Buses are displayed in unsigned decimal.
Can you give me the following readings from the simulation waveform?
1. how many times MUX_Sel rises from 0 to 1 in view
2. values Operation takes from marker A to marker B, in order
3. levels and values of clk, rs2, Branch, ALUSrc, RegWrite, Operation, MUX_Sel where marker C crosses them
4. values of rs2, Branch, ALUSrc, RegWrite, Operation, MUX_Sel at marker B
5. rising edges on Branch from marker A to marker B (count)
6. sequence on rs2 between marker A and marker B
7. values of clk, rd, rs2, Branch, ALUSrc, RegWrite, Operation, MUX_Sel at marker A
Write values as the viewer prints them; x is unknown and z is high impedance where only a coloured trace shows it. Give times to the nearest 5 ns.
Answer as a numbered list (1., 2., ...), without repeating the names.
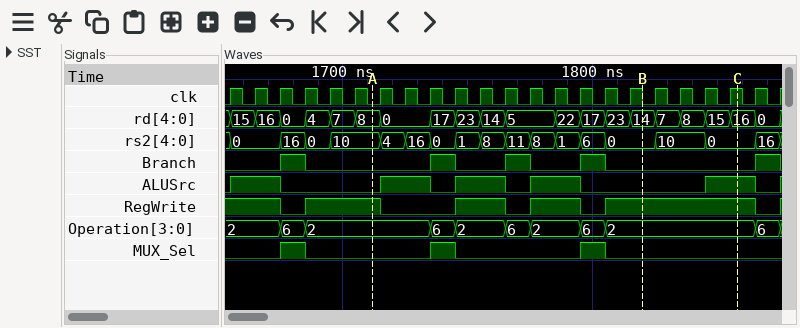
1. 3
2. 2, 6, 2, 6, 2, 6, 2
3. clk=1, rs2=0, Branch=0, ALUSrc=1, RegWrite=1, Operation=2, MUX_Sel=0
4. rs2=0, Branch=0, ALUSrc=0, RegWrite=1, Operation=2, MUX_Sel=0
5. 3
6. 10, 4, 16, 0, 1, 8, 11, 8, 1, 6, 0
7. clk=0, rd=8, rs2=10, Branch=0, ALUSrc=0, RegWrite=1, Operation=2, MUX_Sel=0
